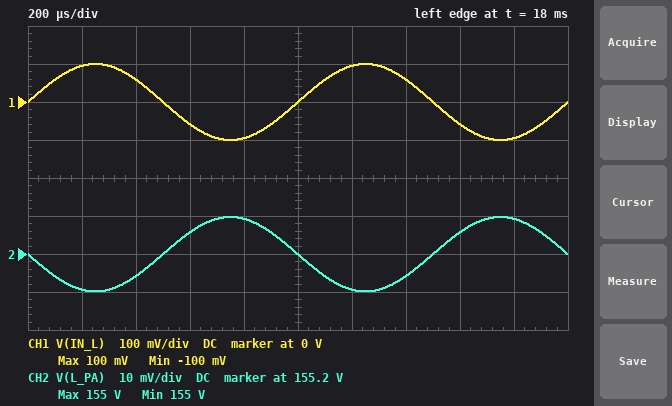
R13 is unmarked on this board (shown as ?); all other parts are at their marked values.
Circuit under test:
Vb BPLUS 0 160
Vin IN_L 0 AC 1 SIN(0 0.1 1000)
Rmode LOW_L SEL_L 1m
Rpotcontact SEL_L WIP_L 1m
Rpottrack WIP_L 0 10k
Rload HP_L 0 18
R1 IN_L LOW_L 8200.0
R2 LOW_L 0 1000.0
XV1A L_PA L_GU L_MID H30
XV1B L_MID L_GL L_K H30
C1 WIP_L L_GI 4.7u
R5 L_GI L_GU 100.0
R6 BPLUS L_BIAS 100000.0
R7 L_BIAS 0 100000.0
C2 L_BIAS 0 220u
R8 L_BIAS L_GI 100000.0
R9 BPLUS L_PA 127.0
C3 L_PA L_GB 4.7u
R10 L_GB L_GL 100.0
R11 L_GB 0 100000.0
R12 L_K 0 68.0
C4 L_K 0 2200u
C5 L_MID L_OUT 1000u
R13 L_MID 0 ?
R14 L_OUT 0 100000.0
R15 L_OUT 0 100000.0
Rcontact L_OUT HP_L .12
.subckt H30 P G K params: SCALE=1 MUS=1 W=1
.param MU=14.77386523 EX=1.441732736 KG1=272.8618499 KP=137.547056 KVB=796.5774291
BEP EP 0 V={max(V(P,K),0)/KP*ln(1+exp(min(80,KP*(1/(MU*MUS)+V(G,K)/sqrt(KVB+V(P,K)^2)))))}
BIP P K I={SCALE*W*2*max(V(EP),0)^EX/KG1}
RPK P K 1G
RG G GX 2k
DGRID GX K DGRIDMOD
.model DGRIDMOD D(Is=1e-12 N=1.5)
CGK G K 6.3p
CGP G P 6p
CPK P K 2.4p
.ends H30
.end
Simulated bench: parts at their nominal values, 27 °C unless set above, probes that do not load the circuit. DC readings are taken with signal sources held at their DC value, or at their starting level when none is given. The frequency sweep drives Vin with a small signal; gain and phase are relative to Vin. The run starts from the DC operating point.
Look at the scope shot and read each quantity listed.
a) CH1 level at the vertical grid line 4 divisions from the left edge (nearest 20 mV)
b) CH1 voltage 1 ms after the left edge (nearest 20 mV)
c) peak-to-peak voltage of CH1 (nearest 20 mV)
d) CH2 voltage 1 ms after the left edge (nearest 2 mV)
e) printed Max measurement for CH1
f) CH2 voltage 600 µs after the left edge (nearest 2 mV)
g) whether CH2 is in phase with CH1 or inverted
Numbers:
-100 mV
0 V
200 mV
155.180 V
100 mV
155.186 V
inverted
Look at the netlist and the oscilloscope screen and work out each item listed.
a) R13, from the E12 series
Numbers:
56 kΩ
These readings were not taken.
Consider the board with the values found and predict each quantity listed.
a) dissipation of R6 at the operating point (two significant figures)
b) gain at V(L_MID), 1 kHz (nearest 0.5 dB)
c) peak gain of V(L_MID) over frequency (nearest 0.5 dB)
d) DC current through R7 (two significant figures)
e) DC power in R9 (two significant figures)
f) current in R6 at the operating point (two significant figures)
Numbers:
64 mW
-27.5 dB
-22.0 dB
800 µA
180 mW
800 µA
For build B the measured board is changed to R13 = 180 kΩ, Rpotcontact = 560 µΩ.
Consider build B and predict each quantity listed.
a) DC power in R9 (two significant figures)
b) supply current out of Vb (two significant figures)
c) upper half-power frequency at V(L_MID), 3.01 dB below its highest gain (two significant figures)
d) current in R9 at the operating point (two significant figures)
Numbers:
170 mW
38 mA
7.2 Hz
37 mA
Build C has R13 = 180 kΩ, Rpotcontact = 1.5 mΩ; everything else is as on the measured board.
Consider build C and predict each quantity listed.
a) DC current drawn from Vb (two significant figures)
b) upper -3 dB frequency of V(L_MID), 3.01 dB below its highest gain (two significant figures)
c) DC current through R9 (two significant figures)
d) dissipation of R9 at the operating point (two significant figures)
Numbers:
38 mA
7.2 Hz
37 mA
170 mW
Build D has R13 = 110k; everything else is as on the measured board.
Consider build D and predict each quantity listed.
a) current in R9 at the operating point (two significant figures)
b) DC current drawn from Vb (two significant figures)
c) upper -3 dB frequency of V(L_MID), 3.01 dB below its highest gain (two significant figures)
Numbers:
37 mA
38 mA
7.2 Hz
